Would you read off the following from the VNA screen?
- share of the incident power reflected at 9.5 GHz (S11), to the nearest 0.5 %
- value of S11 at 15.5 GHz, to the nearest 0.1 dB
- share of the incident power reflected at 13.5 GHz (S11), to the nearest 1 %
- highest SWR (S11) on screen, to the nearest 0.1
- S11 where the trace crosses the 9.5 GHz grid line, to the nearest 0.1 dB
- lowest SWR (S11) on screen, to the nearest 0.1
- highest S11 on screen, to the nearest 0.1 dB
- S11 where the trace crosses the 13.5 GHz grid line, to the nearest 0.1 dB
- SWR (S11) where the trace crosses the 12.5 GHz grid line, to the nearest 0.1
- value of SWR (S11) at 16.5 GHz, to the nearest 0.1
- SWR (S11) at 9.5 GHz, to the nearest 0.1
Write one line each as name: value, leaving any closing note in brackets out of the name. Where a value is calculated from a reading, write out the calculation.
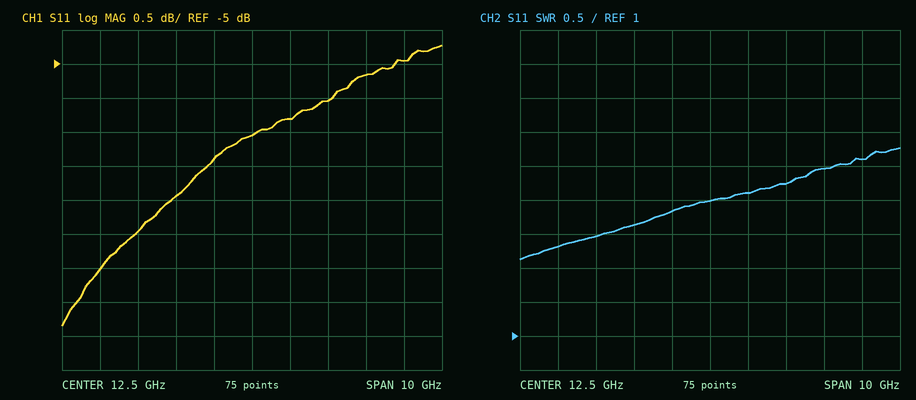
share of the incident power reflected at 9.5 GHz (S11), to the nearest 0.5 %: 10^(-7.5/10) ≈ 17.8 %, so 18.0 % to the nearest 0.5 %
value of S11 at 15.5 GHz, to the nearest 0.1 dB: -5.2 dB
share of the incident power reflected at 13.5 GHz (S11), to the nearest 1 %: 10^(-5.8/10) ≈ 26 %
highest SWR (S11) on screen, to the nearest 0.1: 3.8
S11 where the trace crosses the 9.5 GHz grid line, to the nearest 0.1 dB: -7.5 dB
lowest SWR (S11) on screen, to the nearest 0.1: 2.1
highest S11 on screen, to the nearest 0.1 dB: -4.7 dB
S11 where the trace crosses the 13.5 GHz grid line, to the nearest 0.1 dB: -5.8 dB
SWR (S11) where the trace crosses the 12.5 GHz grid line, to the nearest 0.1: 3.0
value of SWR (S11) at 16.5 GHz, to the nearest 0.1: 3.6
SWR (S11) at 9.5 GHz, to the nearest 0.1: 2.5
